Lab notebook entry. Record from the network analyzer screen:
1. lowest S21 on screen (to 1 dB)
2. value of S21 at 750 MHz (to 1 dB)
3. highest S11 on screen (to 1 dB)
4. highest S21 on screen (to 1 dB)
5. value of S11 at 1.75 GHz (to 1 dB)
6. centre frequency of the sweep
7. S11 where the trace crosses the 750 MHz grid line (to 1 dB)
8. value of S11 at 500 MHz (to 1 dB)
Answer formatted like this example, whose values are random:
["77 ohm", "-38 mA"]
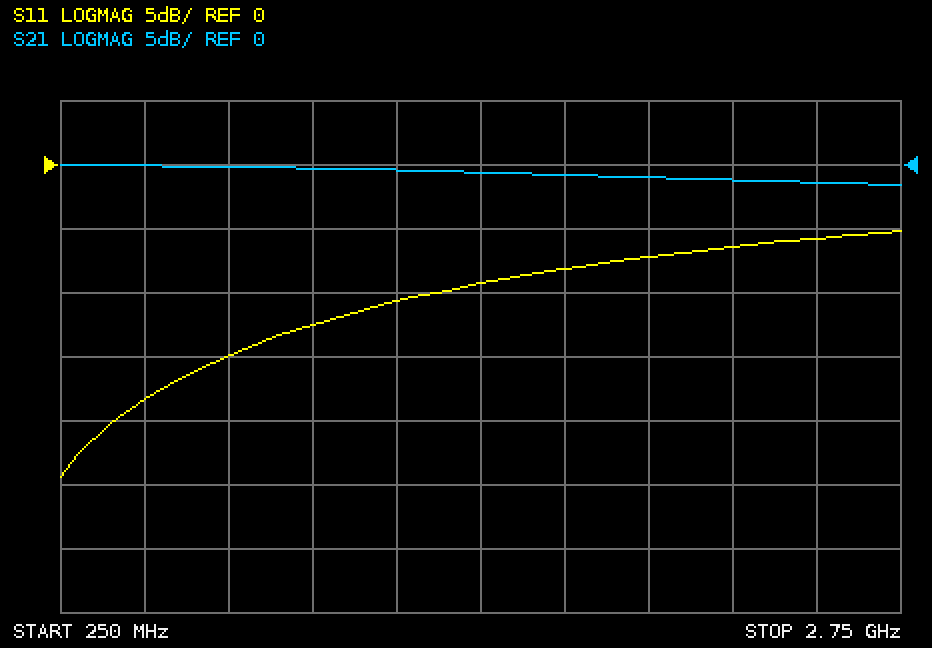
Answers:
["-2 dB", "0 dB", "-5 dB", "0 dB", "-8 dB", "1.5 GHz", "-15 dB", "-18 dB"]
